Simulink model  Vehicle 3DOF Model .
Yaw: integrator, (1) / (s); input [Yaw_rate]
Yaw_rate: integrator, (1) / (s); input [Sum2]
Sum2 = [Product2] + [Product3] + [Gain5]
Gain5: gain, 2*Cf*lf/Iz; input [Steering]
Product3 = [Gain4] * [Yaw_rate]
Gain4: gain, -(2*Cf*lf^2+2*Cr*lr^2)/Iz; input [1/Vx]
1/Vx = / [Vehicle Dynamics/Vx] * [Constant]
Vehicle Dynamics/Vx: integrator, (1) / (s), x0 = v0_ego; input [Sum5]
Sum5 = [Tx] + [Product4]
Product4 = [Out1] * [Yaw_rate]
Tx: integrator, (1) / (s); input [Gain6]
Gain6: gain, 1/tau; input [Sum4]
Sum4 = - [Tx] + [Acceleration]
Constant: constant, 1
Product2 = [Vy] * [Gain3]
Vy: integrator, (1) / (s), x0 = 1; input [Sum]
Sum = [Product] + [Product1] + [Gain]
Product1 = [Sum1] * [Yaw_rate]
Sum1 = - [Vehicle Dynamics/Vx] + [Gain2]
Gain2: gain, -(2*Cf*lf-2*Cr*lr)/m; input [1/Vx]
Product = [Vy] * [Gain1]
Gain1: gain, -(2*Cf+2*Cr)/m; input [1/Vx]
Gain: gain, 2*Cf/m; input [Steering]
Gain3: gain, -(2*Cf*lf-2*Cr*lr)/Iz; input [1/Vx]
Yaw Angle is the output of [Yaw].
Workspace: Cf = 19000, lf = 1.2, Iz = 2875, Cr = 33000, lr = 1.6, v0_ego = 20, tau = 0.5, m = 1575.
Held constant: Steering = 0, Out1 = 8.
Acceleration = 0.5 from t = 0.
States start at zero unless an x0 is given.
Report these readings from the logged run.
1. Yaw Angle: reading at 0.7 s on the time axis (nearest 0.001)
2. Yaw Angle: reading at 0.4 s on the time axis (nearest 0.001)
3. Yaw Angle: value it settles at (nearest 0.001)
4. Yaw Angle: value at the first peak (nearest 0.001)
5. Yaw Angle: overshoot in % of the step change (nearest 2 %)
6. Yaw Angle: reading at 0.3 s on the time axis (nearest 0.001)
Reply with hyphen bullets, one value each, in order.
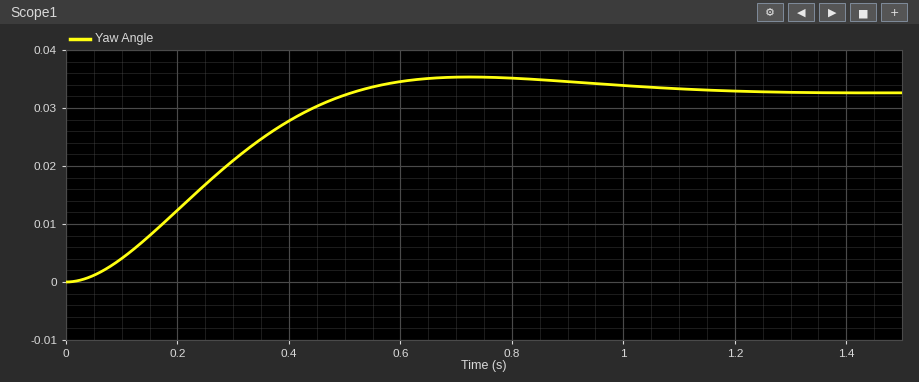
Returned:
- 0.035
- 0.028
- 0.033
- 0.035
- 8 %
- 0.021
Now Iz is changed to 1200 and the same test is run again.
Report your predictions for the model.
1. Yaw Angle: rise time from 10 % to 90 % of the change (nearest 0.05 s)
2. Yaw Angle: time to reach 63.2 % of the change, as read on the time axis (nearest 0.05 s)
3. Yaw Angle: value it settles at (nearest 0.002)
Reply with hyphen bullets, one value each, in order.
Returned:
- 0.25 s
- 0.20 s
- 0.032
